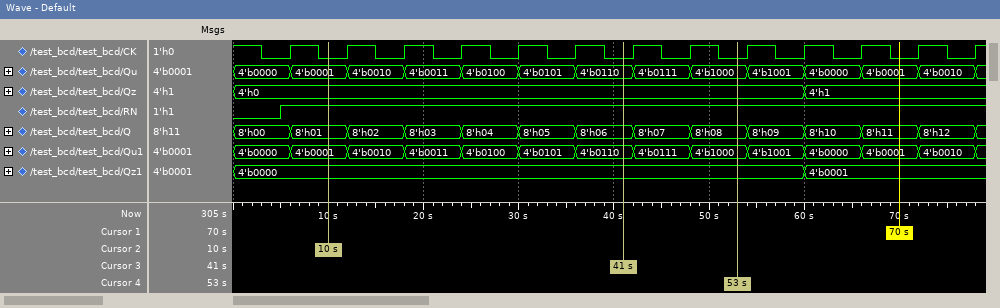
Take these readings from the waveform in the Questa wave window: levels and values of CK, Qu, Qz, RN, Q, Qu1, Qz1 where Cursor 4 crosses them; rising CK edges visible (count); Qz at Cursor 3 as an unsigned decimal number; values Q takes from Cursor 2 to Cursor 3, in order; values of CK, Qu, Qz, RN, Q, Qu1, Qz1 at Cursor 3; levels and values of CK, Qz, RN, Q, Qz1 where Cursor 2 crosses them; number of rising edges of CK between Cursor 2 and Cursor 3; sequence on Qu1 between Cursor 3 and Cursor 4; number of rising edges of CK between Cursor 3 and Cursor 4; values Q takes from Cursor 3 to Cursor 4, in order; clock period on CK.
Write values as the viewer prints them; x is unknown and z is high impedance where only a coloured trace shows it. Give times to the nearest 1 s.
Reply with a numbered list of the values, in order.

1. CK=0, Qu=4'b1000, Qz=4'h0, RN=1, Q=8'h08, Qu1=4'b1000, Qz1=4'b0000
2. 13
3. 0
4. 8'h01, 8'h02, 8'h03, 8'h04, 8'h05, 8'h06
5. CK=0, Qu=4'b0110, Qz=4'h0, RN=1, Q=8'h06, Qu1=4'b0110, Qz1=4'b0000
6. CK=0, Qz=4'h0, RN=1, Q=8'h01, Qz1=4'b0000
7. 5
8. 4'b0110, 4'b0111, 4'b1000
9. 2
10. 8'h06, 8'h07, 8'h08
11. 6 s
